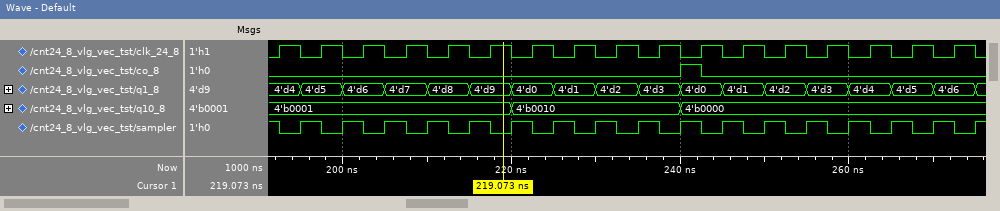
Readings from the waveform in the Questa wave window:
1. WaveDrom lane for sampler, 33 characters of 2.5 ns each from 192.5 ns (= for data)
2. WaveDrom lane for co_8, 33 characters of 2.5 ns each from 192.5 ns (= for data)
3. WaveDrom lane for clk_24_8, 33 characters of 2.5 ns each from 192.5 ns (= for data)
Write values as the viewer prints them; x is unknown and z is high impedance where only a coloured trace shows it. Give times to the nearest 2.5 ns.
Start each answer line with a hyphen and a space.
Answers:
- {name: 'sampler', wave: '010101010101010101010101010101010'}
- {name: 'co_8', wave: '0..................10............'}
- {name: 'clk_24_8', wave: '101010101010101010101010101010101'}
